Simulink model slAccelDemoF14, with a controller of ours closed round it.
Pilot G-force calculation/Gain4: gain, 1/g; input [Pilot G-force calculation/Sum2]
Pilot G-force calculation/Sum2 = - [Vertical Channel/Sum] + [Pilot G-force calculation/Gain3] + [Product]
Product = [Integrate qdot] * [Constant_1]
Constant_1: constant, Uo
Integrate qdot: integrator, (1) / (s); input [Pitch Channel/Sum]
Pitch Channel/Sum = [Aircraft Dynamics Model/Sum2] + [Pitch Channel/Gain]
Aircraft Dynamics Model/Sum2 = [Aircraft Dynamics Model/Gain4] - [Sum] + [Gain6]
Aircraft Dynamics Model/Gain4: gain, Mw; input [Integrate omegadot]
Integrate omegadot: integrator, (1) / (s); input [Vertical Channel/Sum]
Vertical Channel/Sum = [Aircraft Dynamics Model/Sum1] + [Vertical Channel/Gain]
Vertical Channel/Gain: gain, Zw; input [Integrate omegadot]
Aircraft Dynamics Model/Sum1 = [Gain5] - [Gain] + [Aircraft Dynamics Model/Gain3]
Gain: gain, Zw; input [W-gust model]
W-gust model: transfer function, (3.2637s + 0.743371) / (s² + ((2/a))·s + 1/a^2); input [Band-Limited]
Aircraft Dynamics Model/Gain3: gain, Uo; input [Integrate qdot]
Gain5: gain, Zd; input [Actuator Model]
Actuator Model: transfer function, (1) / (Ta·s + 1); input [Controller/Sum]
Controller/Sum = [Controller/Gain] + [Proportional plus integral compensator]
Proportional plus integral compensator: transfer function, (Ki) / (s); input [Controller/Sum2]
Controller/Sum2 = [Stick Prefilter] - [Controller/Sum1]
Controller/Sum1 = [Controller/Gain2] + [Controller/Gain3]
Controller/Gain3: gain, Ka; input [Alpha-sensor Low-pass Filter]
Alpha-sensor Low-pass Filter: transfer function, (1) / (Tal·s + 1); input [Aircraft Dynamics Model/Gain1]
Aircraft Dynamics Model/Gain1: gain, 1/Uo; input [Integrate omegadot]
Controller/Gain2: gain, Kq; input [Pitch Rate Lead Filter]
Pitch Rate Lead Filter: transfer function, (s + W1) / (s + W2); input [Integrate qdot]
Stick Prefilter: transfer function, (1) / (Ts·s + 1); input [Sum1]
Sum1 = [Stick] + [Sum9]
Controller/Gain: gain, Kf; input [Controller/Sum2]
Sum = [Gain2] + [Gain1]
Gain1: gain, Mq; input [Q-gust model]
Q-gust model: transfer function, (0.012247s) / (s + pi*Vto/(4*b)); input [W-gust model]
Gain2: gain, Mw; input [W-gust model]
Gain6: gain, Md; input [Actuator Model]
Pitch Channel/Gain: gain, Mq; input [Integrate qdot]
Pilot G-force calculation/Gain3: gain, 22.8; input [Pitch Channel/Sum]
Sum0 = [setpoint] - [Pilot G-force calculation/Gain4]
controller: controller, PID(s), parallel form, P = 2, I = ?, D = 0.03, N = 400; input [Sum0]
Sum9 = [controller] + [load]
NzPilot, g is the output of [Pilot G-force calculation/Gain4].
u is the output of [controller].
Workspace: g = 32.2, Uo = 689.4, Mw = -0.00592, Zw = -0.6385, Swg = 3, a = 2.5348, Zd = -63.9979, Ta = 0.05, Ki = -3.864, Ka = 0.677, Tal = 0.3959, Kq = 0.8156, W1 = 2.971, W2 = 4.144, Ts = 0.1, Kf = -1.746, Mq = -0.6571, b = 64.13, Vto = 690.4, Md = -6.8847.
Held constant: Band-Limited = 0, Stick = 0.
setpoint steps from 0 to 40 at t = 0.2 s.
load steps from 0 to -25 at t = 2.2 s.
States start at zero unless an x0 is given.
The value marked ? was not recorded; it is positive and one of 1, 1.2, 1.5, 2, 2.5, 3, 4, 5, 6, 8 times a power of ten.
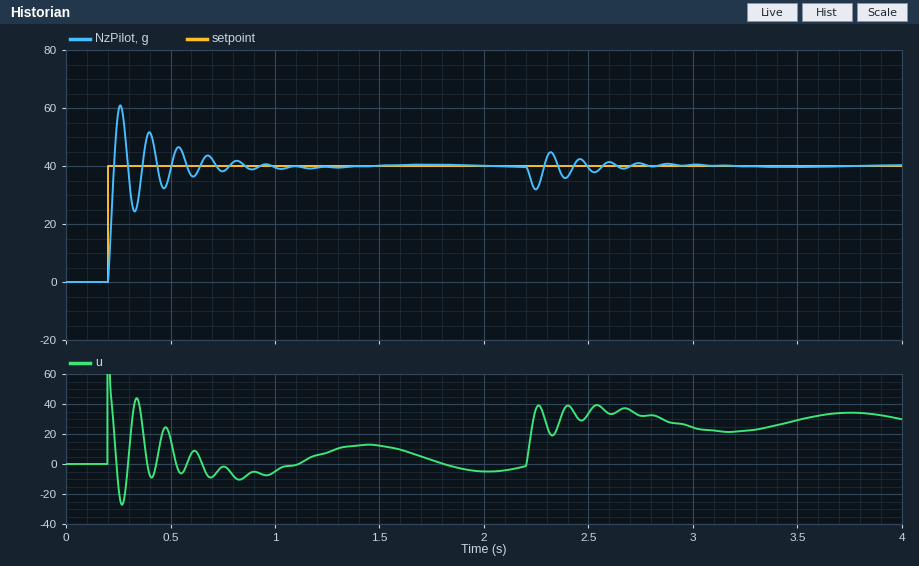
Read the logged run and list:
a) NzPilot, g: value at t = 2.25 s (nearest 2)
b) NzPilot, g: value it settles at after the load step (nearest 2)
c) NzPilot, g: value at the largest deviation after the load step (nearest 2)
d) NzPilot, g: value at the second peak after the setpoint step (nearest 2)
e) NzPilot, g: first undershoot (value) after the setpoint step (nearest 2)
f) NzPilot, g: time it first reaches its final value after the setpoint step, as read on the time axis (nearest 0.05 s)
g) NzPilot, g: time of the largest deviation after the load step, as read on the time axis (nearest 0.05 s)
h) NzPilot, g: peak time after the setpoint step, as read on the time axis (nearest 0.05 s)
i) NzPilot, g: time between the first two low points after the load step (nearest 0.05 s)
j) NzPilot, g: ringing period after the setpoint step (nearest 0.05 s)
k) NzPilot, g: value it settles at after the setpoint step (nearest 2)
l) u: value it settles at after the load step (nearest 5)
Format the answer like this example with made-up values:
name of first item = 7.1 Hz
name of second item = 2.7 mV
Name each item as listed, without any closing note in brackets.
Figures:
NzPilot, g: value at t = 2.25 s = 32
NzPilot, g: value it settles at after the load step = 40
NzPilot, g: value at the largest deviation after the load step = 32
NzPilot, g: value at the second peak after the setpoint step = 52
NzPilot, g: first undershoot (value) after the setpoint step = 24
NzPilot, g: time it first reaches its final value after the setpoint step, as read on the time axis = 0.25 s
NzPilot, g: time of the largest deviation after the load step, as read on the time axis = 2.25 s
NzPilot, g: peak time after the setpoint step, as read on the time axis = 0.25 s
NzPilot, g: time between the first two low points after the load step = 0.15 s
NzPilot, g: ringing period after the setpoint step = 0.15 s
NzPilot, g: value it settles at after the setpoint step = 40
u: value it settles at after the load step = 30
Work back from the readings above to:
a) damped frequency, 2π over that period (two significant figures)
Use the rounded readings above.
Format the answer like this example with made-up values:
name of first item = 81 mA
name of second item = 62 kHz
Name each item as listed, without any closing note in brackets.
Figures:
damped frequency, 2π over that period = 42 rad/s
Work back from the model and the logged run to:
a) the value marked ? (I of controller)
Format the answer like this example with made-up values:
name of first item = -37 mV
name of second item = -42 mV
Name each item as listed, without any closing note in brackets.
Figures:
the value marked ? = 100
